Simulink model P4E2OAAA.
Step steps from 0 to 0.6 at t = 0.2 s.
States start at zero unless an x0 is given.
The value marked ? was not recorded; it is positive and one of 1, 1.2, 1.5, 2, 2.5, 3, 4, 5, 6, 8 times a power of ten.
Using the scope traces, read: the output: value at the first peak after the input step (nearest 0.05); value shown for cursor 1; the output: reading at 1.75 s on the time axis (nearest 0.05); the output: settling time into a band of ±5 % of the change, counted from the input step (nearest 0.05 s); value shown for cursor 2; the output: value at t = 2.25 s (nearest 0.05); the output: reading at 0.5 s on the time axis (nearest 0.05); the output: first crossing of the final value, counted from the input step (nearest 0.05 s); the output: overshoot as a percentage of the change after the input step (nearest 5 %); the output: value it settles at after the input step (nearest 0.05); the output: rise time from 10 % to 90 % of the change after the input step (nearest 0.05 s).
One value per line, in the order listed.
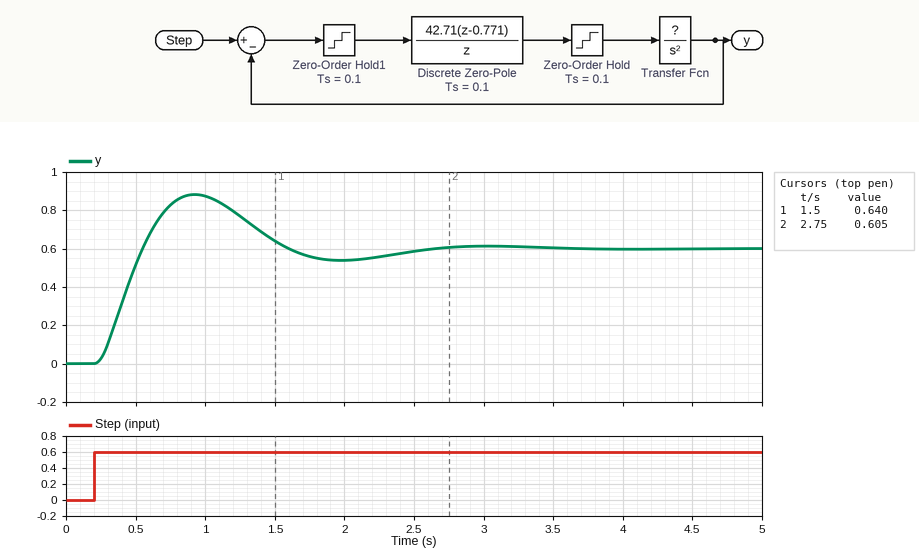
0.90
0.640
0.55
2.15 s
0.605
0.55
0.50
0.35 s
45 %
0.60
0.25 s
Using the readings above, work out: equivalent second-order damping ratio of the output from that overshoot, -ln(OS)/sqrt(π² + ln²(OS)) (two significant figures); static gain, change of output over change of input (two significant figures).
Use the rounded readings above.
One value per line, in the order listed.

0.25
1.0
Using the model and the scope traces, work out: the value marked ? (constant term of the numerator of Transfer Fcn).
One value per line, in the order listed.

0.8
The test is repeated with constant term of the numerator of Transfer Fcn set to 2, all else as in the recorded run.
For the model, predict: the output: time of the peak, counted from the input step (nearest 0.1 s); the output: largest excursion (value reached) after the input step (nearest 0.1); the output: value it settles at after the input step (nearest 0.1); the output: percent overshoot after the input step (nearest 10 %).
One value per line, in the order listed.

0.3 s
1.0
0.6
60 %
